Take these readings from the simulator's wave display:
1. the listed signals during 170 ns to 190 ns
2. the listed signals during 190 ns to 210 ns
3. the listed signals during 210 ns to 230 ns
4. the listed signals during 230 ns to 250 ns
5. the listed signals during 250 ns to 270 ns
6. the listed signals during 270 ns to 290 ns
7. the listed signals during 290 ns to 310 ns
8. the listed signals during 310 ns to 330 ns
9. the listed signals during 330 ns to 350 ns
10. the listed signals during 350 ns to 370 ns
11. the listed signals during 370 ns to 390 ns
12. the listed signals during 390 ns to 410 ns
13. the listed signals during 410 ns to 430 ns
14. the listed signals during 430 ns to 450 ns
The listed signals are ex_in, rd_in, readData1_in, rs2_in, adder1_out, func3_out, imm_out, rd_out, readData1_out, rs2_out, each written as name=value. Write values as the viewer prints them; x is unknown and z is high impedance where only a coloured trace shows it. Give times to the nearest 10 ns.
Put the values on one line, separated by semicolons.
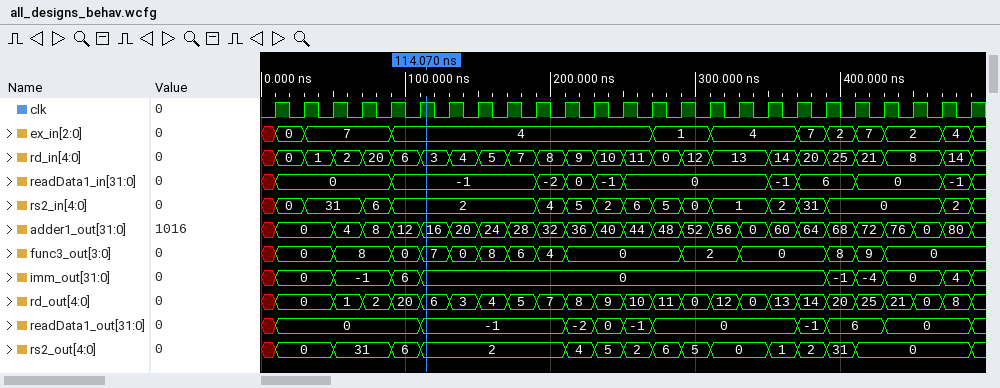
ex_in=4, rd_in=7, readData1_in=-1, rs2_in=2, adder1_out=28, func3_out=6, imm_out=0, rd_out=5, readData1_out=-1, rs2_out=2; ex_in=4, rd_in=8, readData1_in=-2, rs2_in=4, adder1_out=32, func3_out=4, imm_out=0, rd_out=7, readData1_out=-1, rs2_out=2; ex_in=4, rd_in=9, readData1_in=0, rs2_in=5, adder1_out=36, func3_out=0, imm_out=0, rd_out=8, readData1_out=-2, rs2_out=4; ex_in=4, rd_in=10, readData1_in=-1, rs2_in=2, adder1_out=40, func3_out=0, imm_out=0, rd_out=9, readData1_out=0, rs2_out=5; ex_in=4, rd_in=11, readData1_in=0, rs2_in=6, adder1_out=44, func3_out=0, imm_out=0, rd_out=10, readData1_out=-1, rs2_out=2; ex_in=1, rd_in=0, readData1_in=0, rs2_in=5, adder1_out=48, func3_out=0, imm_out=0, rd_out=11, readData1_out=0, rs2_out=6; ex_in=1, rd_in=12, readData1_in=0, rs2_in=0, adder1_out=52, func3_out=2, imm_out=0, rd_out=0, readData1_out=0, rs2_out=5; ex_in=4, rd_in=13, readData1_in=0, rs2_in=1, adder1_out=56, func3_out=2, imm_out=0, rd_out=12, readData1_out=0, rs2_out=0; ex_in=4, rd_in=13, readData1_in=0, rs2_in=1, adder1_out=0, func3_out=0, imm_out=0, rd_out=0, readData1_out=0, rs2_out=0; ex_in=4, rd_in=14, readData1_in=-1, rs2_in=2, adder1_out=60, func3_out=0, imm_out=0, rd_out=13, readData1_out=0, rs2_out=1; ex_in=7, rd_in=20, readData1_in=6, rs2_in=31, adder1_out=64, func3_out=0, imm_out=0, rd_out=14, readData1_out=-1, rs2_out=2; ex_in=2, rd_in=25, readData1_in=6, rs2_in=0, adder1_out=68, func3_out=8, imm_out=-1, rd_out=20, readData1_out=6, rs2_out=31; ex_in=7, rd_in=21, readData1_in=0, rs2_in=0, adder1_out=72, func3_out=9, imm_out=-4, rd_out=25, readData1_out=6, rs2_out=0; ex_in=2, rd_in=8, readData1_in=0, rs2_in=0, adder1_out=76, func3_out=0, imm_out=0, rd_out=21, readData1_out=0, rs2_out=0
